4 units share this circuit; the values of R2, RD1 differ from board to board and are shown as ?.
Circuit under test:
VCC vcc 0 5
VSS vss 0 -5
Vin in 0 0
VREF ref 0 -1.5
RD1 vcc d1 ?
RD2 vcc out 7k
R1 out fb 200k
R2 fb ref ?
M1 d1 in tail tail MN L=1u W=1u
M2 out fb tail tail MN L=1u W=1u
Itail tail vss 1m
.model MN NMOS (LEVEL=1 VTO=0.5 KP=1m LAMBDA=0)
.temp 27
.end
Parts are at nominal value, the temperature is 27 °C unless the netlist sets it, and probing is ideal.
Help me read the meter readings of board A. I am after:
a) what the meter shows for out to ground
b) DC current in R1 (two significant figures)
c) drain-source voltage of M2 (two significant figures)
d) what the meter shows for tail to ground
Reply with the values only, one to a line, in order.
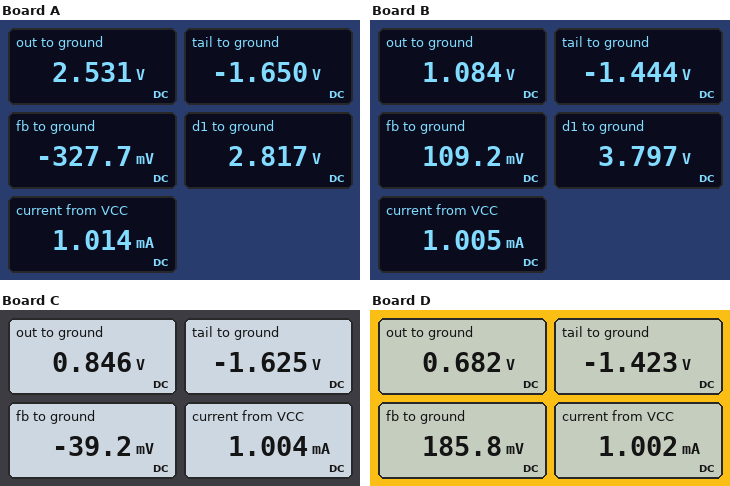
2.531 V
14 µA
4.2 V
-1.650 V
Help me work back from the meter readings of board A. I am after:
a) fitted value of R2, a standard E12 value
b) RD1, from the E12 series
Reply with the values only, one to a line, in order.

82 kΩ
3.3 kΩ
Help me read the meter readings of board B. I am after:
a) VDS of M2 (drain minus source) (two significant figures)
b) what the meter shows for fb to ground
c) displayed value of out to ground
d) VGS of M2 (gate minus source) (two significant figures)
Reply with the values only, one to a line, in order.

2.5 V
109.2 mV
1.084 V
1.6 V
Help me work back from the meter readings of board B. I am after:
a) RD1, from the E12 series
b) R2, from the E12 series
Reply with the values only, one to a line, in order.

2.7 kΩ
330 kΩ
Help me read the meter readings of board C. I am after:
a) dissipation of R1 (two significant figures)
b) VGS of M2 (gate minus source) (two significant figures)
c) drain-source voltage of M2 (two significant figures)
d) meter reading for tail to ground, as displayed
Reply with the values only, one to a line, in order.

3.9 µW
1.6 V
2.5 V
-1.625 V
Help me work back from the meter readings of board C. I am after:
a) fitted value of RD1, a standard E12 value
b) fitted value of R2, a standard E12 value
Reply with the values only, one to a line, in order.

15 kΩ
330 kΩ
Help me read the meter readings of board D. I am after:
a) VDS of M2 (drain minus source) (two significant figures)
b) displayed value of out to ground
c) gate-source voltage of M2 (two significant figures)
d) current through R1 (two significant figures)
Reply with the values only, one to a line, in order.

2.1 V
0.682 V
1.6 V
2.5 µA
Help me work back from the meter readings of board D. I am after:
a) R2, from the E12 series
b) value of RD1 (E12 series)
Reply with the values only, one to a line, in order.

680 kΩ
15 kΩ
